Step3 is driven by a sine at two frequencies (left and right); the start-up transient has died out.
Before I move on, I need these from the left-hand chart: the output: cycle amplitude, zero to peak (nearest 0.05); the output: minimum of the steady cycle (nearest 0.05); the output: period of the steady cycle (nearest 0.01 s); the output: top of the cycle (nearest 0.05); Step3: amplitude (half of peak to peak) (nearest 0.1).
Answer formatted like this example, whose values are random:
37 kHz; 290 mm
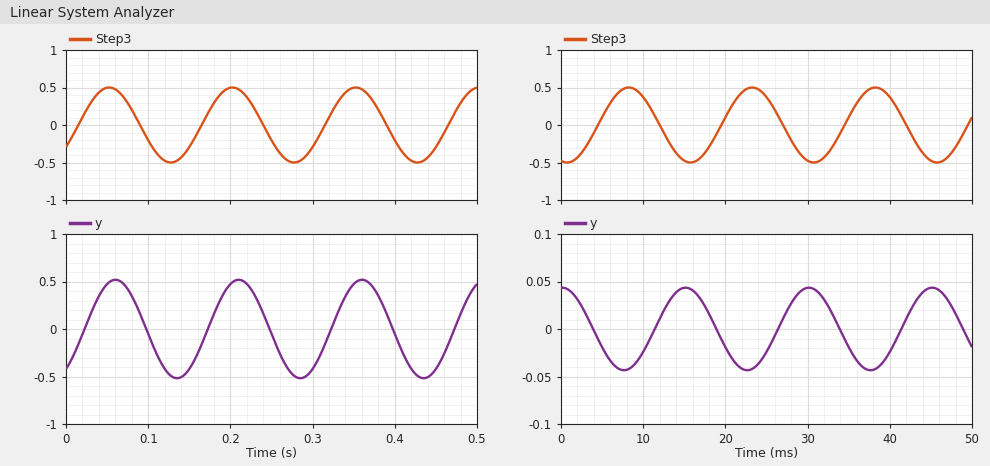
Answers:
0.50; -0.50; 0.15 s; 0.50; 0.5
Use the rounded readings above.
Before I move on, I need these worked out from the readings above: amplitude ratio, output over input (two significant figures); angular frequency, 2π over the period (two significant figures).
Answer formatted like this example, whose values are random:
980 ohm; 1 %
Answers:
1.0; 42 rad/s
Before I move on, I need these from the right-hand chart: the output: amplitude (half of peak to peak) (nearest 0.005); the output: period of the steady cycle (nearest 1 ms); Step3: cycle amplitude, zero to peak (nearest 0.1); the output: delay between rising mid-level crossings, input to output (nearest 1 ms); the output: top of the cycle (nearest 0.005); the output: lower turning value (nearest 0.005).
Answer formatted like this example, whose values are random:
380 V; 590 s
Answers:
0.045; 15 ms; 0.5; 7 ms; 0.045; -0.045
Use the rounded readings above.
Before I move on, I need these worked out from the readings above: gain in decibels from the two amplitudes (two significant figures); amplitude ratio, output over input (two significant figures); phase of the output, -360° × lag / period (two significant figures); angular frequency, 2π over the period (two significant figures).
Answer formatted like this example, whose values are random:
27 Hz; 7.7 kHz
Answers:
-21 dB; 0.090; -170°; 0.42 rad/ms
